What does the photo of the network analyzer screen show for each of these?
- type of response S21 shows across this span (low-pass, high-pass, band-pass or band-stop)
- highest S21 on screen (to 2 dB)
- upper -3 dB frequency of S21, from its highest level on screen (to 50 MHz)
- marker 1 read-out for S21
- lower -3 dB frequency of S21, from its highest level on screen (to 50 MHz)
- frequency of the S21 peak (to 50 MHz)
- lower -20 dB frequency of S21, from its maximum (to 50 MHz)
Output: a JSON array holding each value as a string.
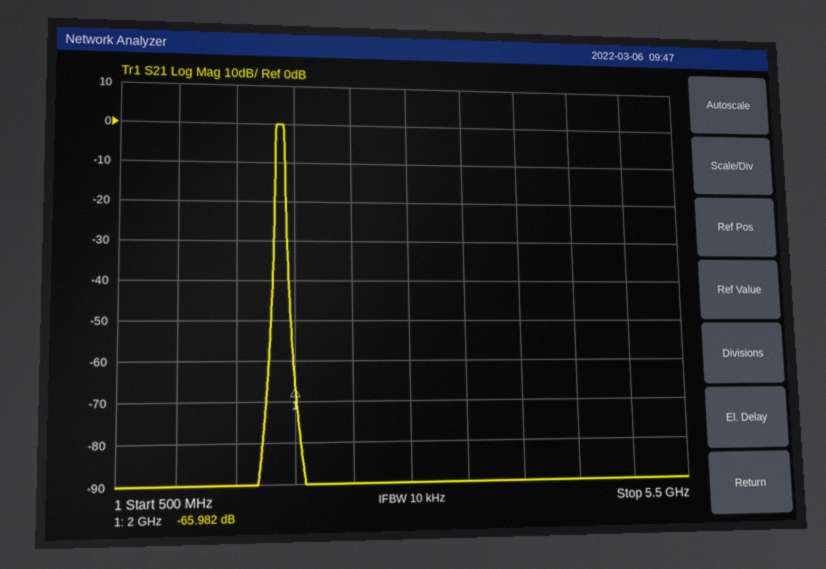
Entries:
["band-pass", "0 dB", "1.90 GHz", "-65.982 dB", "1.85 GHz", "1.85 GHz", "1.85 GHz"]
